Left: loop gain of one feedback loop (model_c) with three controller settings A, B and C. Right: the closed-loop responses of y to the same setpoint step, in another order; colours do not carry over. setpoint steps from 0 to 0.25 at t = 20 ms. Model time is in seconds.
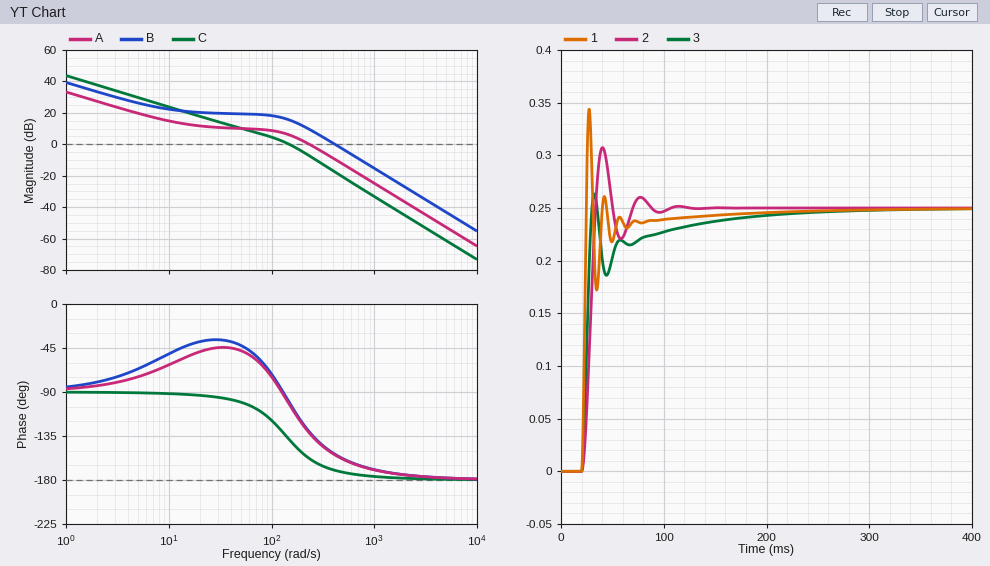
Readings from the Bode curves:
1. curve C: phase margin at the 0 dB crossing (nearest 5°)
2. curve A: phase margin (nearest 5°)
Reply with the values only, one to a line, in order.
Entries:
40°
50°
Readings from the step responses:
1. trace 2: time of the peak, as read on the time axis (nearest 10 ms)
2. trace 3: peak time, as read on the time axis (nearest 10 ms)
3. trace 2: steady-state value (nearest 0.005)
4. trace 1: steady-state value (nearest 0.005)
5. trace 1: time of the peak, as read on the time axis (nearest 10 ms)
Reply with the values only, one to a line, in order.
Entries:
40 ms
30 ms
0.250
0.250
30 ms
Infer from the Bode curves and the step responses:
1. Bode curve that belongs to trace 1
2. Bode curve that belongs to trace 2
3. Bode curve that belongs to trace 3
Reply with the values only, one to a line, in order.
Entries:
B
C
A
